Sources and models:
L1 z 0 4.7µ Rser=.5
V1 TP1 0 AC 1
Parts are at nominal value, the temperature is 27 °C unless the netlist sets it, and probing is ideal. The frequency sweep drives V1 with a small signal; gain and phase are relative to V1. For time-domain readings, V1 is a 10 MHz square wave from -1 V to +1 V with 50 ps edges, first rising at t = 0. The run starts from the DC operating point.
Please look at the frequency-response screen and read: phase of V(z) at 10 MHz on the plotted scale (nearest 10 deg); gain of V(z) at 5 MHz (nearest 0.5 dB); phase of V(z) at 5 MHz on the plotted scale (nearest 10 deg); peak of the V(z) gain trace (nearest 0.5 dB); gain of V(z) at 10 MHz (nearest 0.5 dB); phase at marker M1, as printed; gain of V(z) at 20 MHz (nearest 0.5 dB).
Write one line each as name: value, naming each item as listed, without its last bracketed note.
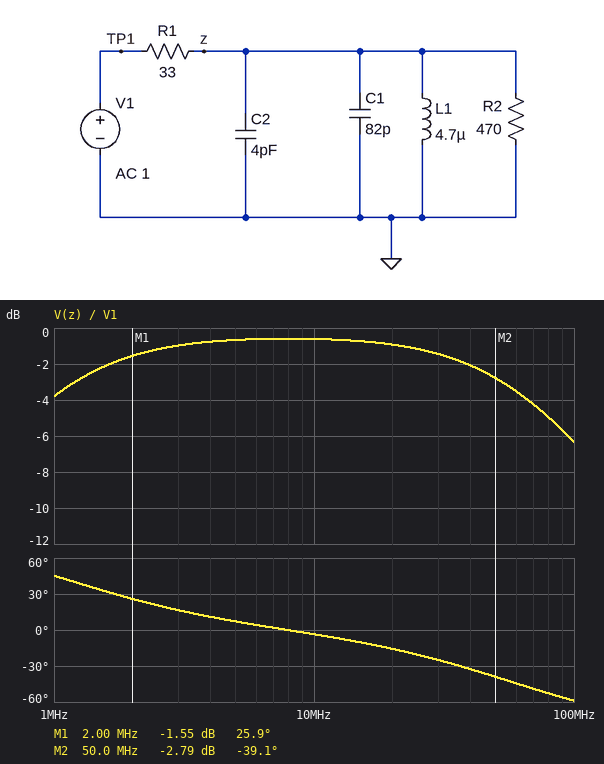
phase of V(z) at 10 MHz on the plotted scale: 0 deg
gain of V(z) at 5 MHz: -0.5 dB
phase of V(z) at 5 MHz on the plotted scale: 10 deg
peak of the V(z) gain trace: -0.5 dB
gain of V(z) at 10 MHz: -0.5 dB
phase at marker M1, as printed: 25.9 deg
gain of V(z) at 20 MHz: -1.0 dB
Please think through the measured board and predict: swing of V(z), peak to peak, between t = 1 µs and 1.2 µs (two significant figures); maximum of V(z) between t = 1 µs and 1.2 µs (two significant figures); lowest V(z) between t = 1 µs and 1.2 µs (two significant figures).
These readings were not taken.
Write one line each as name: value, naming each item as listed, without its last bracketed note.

swing of V(z), peak to peak, between t = 1 µs and 1.2 µs: 2.0 V
maximum of V(z) between t = 1 µs and 1.2 µs: 1.0 V
lowest V(z) between t = 1 µs and 1.2 µs: -1.0 V
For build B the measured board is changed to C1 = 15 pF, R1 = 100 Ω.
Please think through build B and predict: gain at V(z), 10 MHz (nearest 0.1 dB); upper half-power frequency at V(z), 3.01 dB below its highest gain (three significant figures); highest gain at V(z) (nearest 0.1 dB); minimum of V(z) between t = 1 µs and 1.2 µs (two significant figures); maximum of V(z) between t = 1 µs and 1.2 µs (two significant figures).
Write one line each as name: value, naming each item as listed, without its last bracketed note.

gain at V(z), 10 MHz: -1.8 dB
upper half-power frequency at V(z), 3.01 dB below its highest gain: 104 MHz
highest gain at V(z): -1.7 dB
minimum of V(z) between t = 1 µs and 1.2 µs: -1.1 V
maximum of V(z) between t = 1 µs and 1.2 µs: 1.1 V
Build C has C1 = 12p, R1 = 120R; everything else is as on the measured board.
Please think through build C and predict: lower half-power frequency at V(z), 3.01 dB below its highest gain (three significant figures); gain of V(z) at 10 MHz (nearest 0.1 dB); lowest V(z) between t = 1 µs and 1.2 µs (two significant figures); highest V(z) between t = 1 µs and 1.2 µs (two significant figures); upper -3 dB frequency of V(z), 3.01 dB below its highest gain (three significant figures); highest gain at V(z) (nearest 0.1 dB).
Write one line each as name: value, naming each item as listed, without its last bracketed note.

lower half-power frequency at V(z), 3.01 dB below its highest gain: 3.16 MHz
gain of V(z) at 10 MHz: -2.2 dB
lowest V(z) between t = 1 µs and 1.2 µs: -1.1 V
highest V(z) between t = 1 µs and 1.2 µs: 1.1 V
upper -3 dB frequency of V(z), 3.01 dB below its highest gain: 107 MHz
highest gain at V(z): -2.0 dB
